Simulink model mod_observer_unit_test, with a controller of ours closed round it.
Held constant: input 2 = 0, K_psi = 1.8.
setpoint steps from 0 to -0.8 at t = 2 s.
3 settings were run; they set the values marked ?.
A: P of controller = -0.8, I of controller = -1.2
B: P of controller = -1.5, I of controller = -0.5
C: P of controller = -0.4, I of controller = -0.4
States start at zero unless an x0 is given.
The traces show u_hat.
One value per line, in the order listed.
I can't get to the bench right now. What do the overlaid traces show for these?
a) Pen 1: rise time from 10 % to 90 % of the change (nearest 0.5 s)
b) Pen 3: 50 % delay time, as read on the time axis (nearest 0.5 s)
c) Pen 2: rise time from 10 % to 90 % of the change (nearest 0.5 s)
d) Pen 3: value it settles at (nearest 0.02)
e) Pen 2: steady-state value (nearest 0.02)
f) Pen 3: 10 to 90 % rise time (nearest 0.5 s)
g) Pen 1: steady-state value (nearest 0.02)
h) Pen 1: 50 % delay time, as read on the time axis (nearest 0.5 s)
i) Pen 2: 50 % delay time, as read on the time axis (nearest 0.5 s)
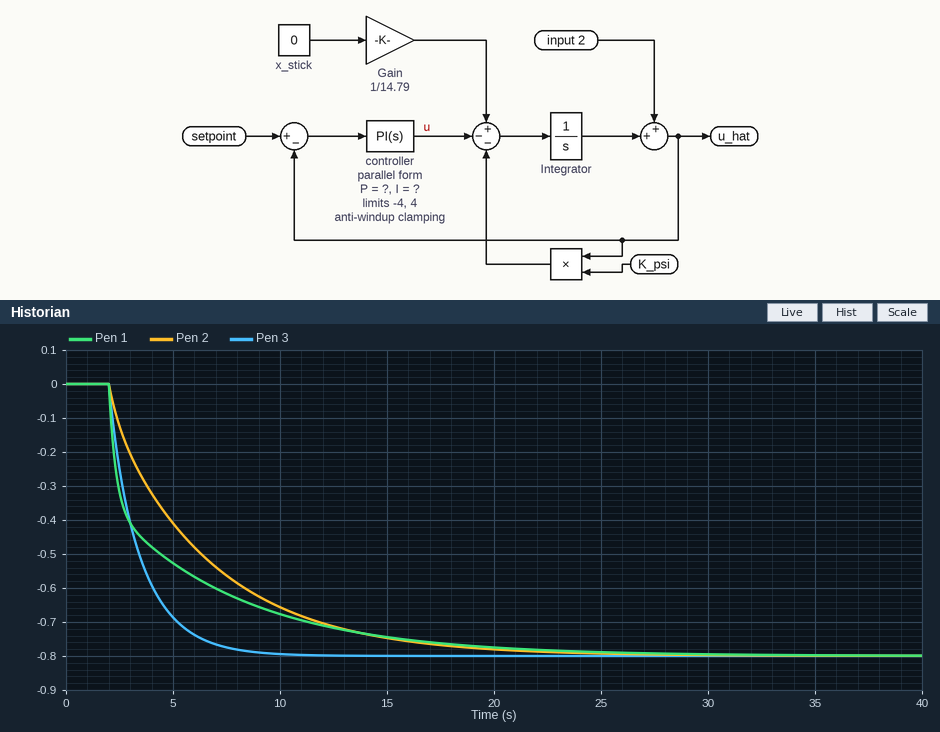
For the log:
10.5 s
3.0 s
10.5 s
-0.80
-0.80
3.5 s
-0.80
3.0 s
5.0 s
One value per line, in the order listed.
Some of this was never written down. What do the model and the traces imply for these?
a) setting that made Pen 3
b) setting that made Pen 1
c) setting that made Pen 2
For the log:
A
B
C
